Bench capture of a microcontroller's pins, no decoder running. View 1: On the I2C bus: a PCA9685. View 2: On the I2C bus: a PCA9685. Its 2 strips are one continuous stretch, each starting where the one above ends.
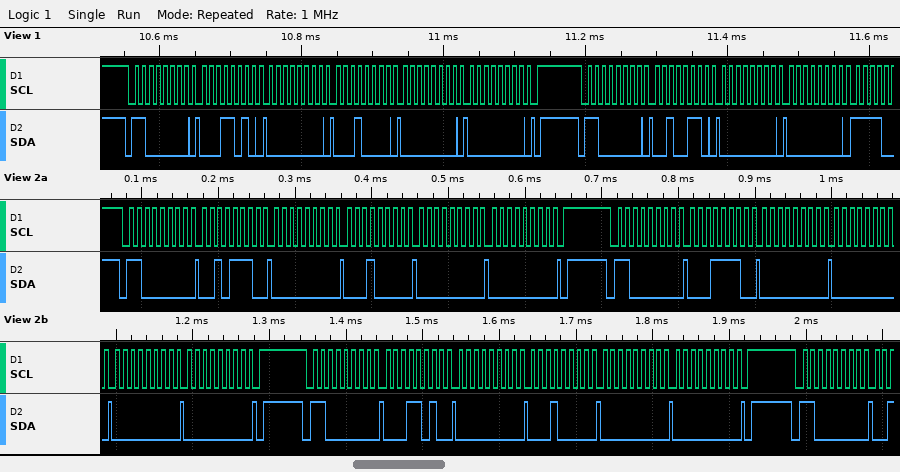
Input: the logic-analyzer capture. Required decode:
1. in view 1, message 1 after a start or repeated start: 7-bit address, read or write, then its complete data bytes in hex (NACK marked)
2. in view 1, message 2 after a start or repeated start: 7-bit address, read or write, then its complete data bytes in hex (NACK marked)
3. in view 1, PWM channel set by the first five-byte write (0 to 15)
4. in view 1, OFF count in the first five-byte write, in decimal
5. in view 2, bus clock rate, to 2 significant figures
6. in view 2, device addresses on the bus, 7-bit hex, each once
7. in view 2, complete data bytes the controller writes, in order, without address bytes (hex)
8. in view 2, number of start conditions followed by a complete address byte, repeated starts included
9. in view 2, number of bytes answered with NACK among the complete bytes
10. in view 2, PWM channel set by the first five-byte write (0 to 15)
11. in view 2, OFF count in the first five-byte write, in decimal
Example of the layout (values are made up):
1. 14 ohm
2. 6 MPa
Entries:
1. 0x60 write: 1A 00 10 00 00
2. 0x60 write: 26 00 00
3. 5
4. 0
5. 100 kHz
6. 0x60
7. 2E 00 10 00 00 1E 00 00 00 00 1A 00 10 00 00
8. 4
9. 0
10. 10
11. 0
